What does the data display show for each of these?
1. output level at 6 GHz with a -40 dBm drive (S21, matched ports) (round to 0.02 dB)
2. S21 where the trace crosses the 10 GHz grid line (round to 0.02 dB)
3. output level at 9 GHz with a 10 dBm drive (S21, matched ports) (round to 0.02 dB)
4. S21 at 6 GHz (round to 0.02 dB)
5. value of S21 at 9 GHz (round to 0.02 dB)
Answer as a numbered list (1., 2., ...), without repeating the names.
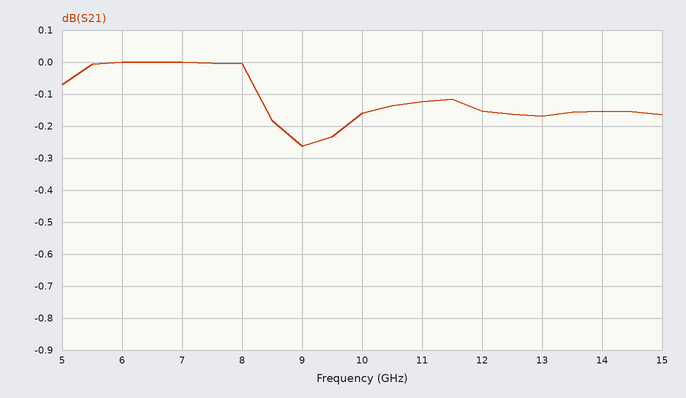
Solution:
1. -40.00 dBm
2. -0.16 dB
3. 9.74 dBm
4. 0.00 dB
5. -0.26 dB
